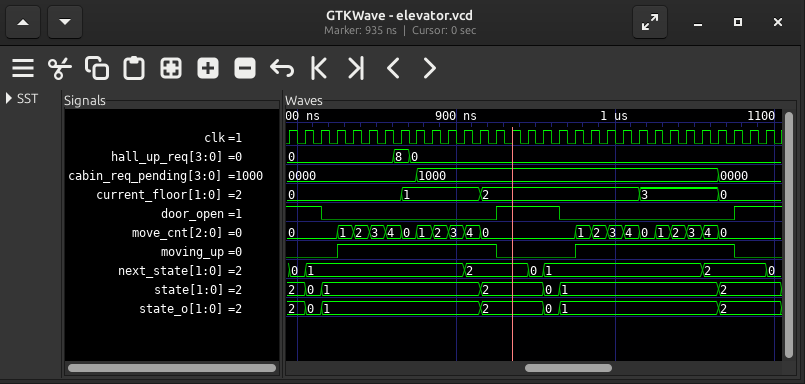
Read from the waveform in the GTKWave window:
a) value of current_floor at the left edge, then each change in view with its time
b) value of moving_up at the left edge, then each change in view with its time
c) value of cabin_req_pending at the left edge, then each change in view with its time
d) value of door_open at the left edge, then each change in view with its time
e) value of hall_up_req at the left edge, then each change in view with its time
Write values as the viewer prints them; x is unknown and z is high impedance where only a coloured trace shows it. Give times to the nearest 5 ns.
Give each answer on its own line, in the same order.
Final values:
0, 1 at 865 ns, 2 at 915 ns, 3 at 1015 ns, 0 at 1065 ns
0, 1 at 825 ns, 0 at 925 ns, 1 at 975 ns, 0 at 1075 ns
0000, 1000 at 875 ns, 0000 at 1065 ns
1, 0 at 815 ns, 1 at 925 ns, 0 at 965 ns, 1 at 1075 ns
0, 8 at 860 ns, 0 at 870 ns
